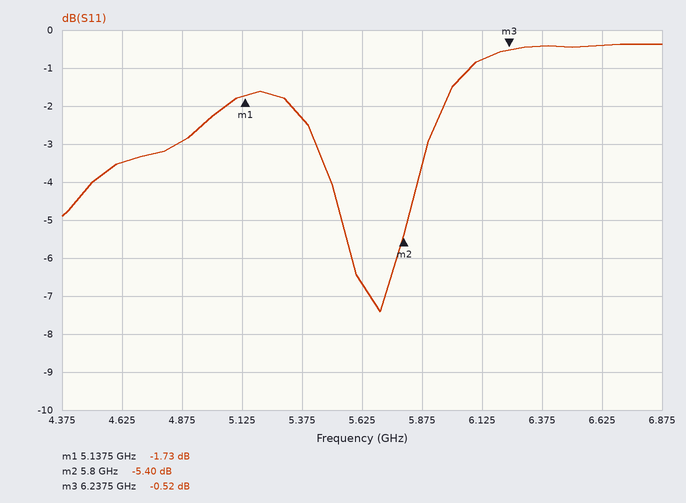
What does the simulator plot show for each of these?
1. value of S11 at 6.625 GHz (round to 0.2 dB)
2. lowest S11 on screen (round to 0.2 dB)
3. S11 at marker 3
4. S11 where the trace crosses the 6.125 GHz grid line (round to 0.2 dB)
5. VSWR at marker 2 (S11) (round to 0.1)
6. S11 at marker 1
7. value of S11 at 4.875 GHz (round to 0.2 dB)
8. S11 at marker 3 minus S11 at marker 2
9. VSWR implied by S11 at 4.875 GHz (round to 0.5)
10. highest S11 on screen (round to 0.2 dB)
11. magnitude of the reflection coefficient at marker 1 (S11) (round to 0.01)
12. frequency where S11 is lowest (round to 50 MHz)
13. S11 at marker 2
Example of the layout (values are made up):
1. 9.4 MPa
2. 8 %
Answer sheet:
1. -0.4 dB
2. -7.4 dB
3. -0.52 dB
4. -0.8 dB
5. 3.3
6. -1.73 dB
7. -3.0 dB
8. 4.88 dB
9. 6.0
10. -0.4 dB
11. 0.82
12. 5.70 GHz
13. -5.40 dB
